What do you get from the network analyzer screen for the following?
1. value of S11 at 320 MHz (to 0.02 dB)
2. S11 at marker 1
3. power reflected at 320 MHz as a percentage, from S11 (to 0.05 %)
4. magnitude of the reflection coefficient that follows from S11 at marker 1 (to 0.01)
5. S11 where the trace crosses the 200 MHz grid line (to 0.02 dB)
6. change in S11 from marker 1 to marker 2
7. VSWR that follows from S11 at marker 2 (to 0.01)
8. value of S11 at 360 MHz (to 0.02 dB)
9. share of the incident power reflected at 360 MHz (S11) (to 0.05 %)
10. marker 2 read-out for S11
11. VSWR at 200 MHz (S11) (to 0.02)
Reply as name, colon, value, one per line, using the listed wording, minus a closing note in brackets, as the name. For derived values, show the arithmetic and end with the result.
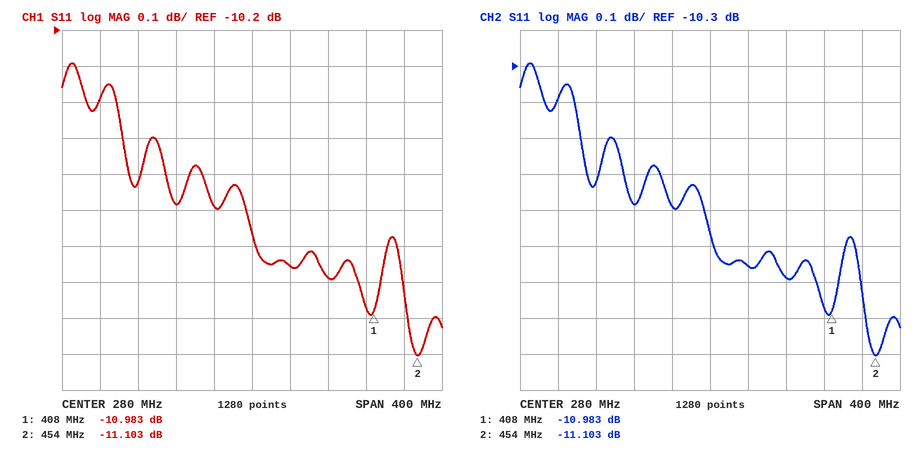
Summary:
value of S11 at 320 MHz: -10.86 dB
S11 at marker 1: -10.983 dB
power reflected at 320 MHz as a percentage, from S11: 10^(-10.86/10) ≈ 8.20 %
magnitude of the reflection coefficient that follows from S11 at marker 1: 10^(-10.983/20) ≈ 0.28
S11 where the trace crosses the 200 MHz grid line: -10.68 dB
change in S11 from marker 1 to marker 2: -11.103 − (-10.983) = -0.120 dB
VSWR that follows from S11 at marker 2: (1 + 0.2785)/(1 − 0.2785) ≈ 1.77
value of S11 at 360 MHz: -10.88 dB
share of the incident power reflected at 360 MHz (S11): 10^(-10.88/10) ≈ 8.17 %, so 8.15 % to the nearest 0.05 %
marker 2 read-out for S11: -11.103 dB
VSWR at 200 MHz (S11): |Γ| = 10^(-10.68/20) = 0.2924; VSWR = (1 + 0.2924)/(1 − 0.2924) ≈ 1.83, so 1.82 to the nearest 0.02
